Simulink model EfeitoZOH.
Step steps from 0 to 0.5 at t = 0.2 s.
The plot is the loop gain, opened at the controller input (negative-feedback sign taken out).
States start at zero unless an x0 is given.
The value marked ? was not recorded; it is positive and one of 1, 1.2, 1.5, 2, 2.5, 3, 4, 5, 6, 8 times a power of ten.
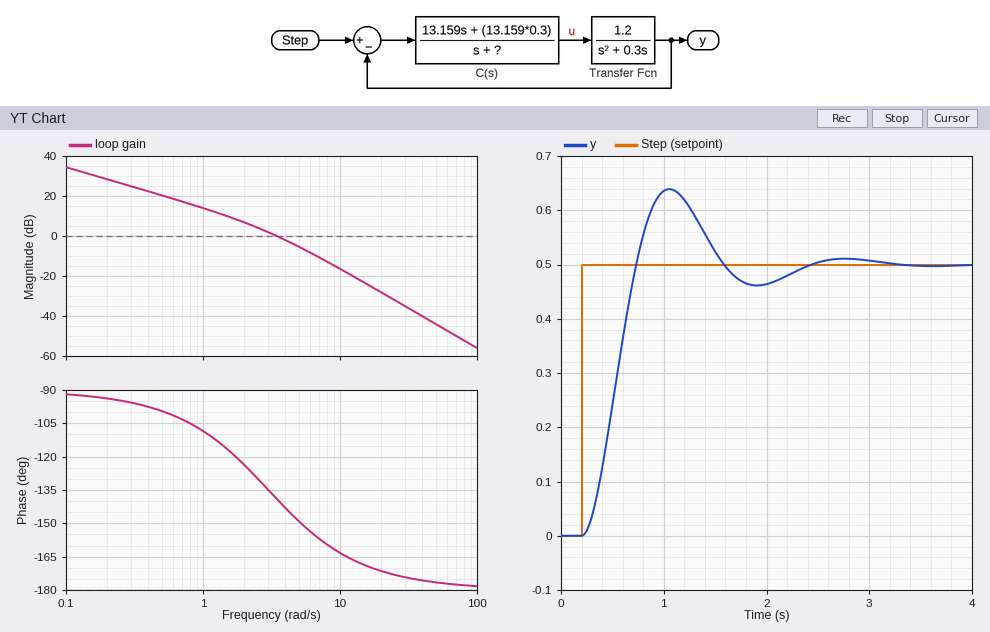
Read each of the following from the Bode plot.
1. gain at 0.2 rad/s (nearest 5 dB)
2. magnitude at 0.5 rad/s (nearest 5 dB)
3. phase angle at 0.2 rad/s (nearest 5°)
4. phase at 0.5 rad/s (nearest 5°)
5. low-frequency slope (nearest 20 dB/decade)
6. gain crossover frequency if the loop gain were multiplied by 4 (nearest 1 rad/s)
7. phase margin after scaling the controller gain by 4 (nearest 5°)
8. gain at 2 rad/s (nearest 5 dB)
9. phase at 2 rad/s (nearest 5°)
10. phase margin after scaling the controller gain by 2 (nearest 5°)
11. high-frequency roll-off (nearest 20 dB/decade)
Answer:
30 dB
20 dB
-95°
-100°
-20 dB/decade
8 rad/s
20°
5 dB
-125°
30°
-40 dB/decade
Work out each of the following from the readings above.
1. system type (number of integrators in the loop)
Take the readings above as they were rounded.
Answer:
1
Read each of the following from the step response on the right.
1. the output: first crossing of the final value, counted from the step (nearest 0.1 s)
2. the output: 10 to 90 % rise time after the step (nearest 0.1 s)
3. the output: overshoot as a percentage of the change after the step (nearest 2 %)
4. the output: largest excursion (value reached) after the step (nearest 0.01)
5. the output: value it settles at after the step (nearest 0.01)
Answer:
0.5 s
0.4 s
28 %
0.64
0.50
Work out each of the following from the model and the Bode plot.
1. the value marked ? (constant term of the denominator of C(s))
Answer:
3
